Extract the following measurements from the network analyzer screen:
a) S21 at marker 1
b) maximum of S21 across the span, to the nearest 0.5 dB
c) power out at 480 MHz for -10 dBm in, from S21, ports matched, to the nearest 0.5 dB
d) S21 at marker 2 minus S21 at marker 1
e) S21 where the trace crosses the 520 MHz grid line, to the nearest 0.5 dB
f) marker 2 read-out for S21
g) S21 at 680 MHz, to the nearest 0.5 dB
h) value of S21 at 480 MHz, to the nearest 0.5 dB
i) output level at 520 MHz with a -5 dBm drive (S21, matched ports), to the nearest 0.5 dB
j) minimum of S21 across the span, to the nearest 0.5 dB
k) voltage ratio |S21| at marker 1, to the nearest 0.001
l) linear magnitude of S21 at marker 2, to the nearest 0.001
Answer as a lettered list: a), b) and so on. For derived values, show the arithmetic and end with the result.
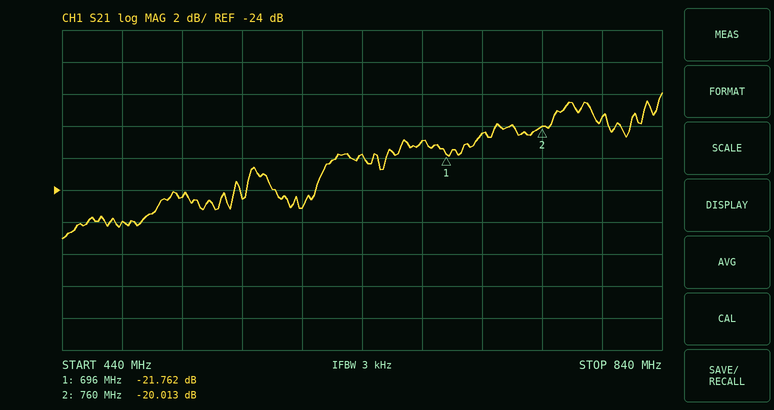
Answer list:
a) -21.762 dB
b) -18.0 dB
c) -10 dBm + (-26.0 dB) = -36.0 dBm
d) -20.013 − (-21.762) = 1.749 dB
e) -24.5 dB
f) -20.013 dB
g) -21.0 dB
h) -26.0 dB
i) -5 dBm + (-24.5 dB) = -29.5 dBm
j) -27.0 dB
k) 10^(-21.762/20) ≈ 0.082
l) 10^(-20.013/20) ≈ 0.100
